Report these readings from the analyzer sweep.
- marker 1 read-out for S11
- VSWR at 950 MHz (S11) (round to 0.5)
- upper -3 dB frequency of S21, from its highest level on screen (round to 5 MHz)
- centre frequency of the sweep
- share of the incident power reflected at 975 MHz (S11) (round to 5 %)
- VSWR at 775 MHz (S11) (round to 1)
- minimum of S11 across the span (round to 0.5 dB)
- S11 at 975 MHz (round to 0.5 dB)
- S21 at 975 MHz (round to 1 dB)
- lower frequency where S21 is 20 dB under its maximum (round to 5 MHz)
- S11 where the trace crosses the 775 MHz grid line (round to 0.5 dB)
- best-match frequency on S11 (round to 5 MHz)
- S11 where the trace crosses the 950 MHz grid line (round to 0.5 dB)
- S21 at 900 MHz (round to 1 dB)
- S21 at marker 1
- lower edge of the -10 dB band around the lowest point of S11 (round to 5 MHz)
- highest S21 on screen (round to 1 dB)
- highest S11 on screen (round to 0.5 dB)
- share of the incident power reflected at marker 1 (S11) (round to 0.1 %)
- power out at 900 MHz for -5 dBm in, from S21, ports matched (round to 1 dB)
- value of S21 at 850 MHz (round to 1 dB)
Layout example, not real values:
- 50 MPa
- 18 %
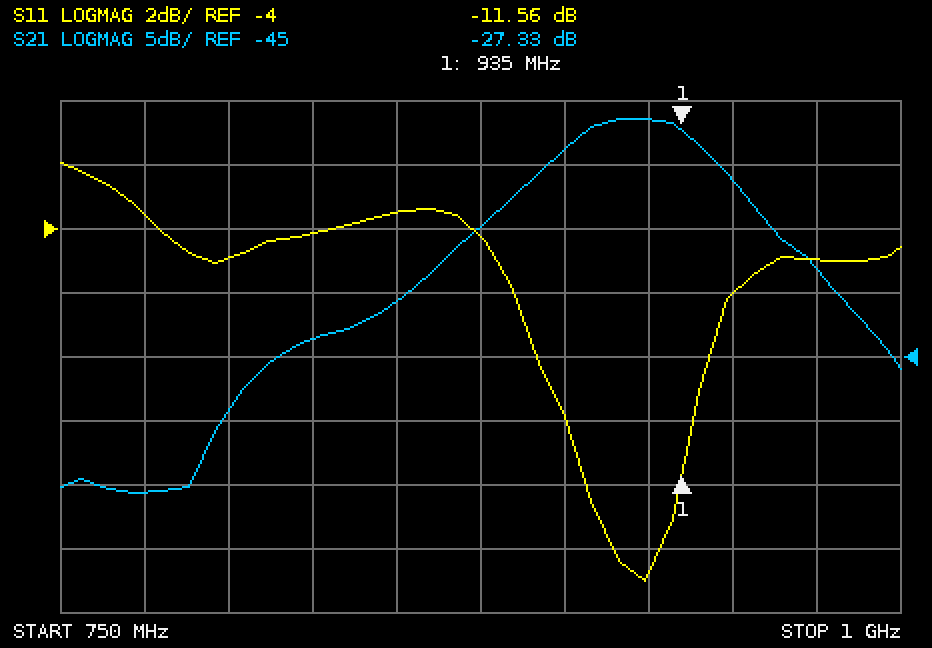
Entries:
- -11.56 dB
- 3.0
- 945 MHz
- 875 MHz
- 30 %
- 5
- -15.0 dB
- -5.0 dB
- -38 dB
- 810 MHz
- -3.5 dB
- 925 MHz
- -6.0 dB
- -29 dB
- -27.33 dB
- 900 MHz
- -26 dB
- -2.0 dB
- 7.0 %
- -34 dBm
- -41 dB
